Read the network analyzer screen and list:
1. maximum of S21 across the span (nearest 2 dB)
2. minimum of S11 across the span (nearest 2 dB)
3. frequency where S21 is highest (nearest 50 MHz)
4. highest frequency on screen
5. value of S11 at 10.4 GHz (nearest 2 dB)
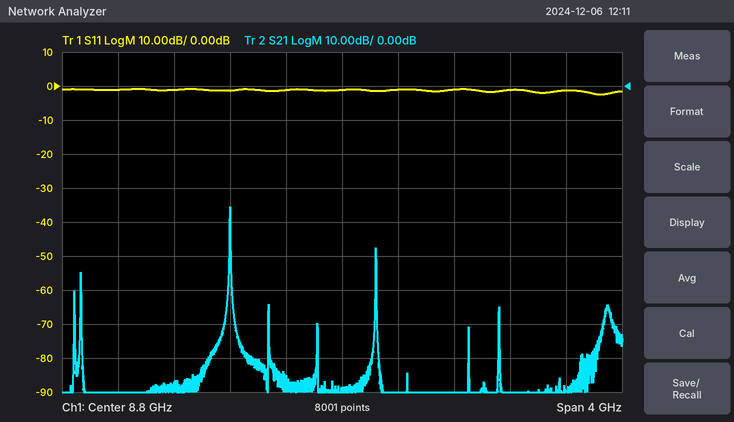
-36 dB
-2 dB
8.00 GHz
10.8 GHz
-2 dB
